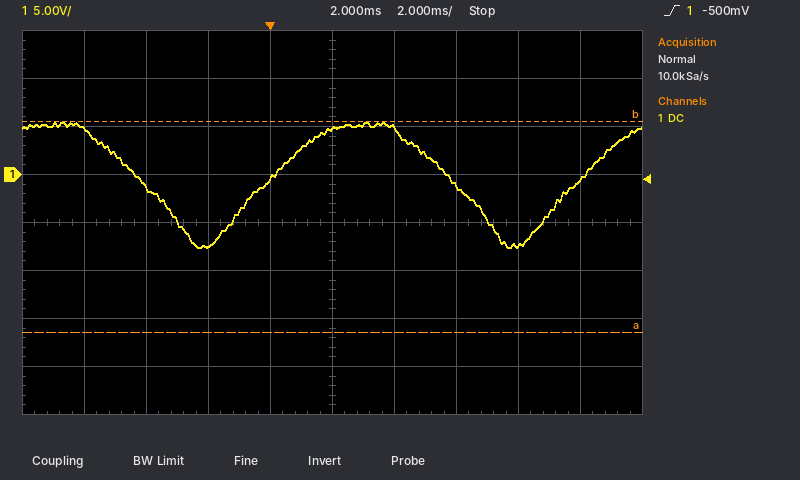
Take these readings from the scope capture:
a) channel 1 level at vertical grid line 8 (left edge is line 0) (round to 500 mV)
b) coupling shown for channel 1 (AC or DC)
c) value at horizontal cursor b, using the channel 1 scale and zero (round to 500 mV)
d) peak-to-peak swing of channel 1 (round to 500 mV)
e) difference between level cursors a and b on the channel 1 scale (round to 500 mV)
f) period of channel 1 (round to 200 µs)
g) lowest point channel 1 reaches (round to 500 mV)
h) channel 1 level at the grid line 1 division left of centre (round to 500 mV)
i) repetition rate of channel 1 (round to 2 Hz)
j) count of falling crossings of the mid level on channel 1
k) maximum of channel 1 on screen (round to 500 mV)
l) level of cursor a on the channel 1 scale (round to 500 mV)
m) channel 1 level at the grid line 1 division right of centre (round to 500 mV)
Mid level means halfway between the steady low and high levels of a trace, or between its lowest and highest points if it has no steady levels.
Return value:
-7.5 V
DC
5.5 V
13.0 V
22.0 V
10.0 ms
-7.5 V
-500 mV
100 Hz
2
5.5 V
-16.5 V
5.0 V
